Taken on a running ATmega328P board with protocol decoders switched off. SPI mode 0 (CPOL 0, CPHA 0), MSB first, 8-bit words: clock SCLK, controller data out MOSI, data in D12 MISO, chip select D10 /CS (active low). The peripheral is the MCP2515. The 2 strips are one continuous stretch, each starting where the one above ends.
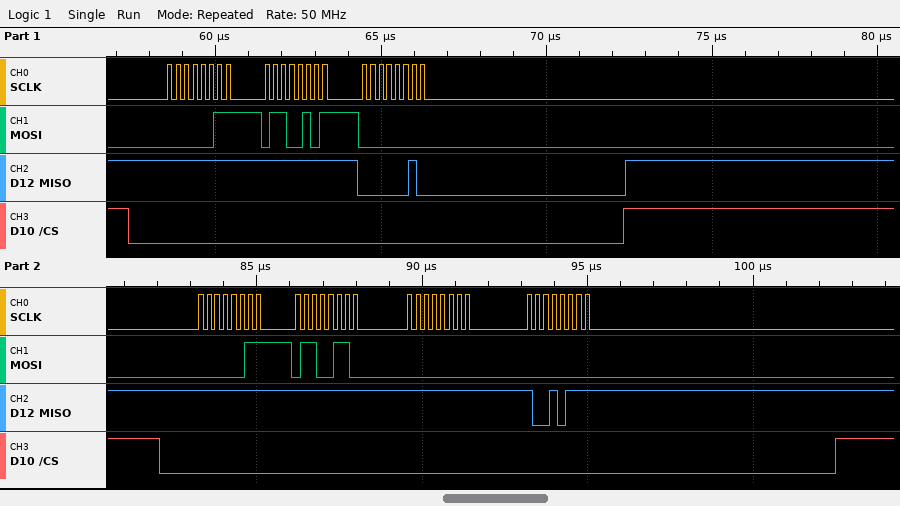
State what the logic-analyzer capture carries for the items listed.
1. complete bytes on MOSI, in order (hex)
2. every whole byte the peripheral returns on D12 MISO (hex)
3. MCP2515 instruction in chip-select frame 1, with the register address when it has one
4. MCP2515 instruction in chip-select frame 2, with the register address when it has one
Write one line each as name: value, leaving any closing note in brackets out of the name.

complete bytes on MOSI, in order: 0x03 0x65 0x00 0x03 0x66 0x00 0x00
every whole byte the peripheral returns on D12 MISO: 0xFF 0xFF 0x02 0xFF 0xFF 0xFF 0x97
MCP2515 instruction in chip-select frame 1, with the register address when it has one: READ 0x65
MCP2515 instruction in chip-select frame 2, with the register address when it has one: READ 0x66
